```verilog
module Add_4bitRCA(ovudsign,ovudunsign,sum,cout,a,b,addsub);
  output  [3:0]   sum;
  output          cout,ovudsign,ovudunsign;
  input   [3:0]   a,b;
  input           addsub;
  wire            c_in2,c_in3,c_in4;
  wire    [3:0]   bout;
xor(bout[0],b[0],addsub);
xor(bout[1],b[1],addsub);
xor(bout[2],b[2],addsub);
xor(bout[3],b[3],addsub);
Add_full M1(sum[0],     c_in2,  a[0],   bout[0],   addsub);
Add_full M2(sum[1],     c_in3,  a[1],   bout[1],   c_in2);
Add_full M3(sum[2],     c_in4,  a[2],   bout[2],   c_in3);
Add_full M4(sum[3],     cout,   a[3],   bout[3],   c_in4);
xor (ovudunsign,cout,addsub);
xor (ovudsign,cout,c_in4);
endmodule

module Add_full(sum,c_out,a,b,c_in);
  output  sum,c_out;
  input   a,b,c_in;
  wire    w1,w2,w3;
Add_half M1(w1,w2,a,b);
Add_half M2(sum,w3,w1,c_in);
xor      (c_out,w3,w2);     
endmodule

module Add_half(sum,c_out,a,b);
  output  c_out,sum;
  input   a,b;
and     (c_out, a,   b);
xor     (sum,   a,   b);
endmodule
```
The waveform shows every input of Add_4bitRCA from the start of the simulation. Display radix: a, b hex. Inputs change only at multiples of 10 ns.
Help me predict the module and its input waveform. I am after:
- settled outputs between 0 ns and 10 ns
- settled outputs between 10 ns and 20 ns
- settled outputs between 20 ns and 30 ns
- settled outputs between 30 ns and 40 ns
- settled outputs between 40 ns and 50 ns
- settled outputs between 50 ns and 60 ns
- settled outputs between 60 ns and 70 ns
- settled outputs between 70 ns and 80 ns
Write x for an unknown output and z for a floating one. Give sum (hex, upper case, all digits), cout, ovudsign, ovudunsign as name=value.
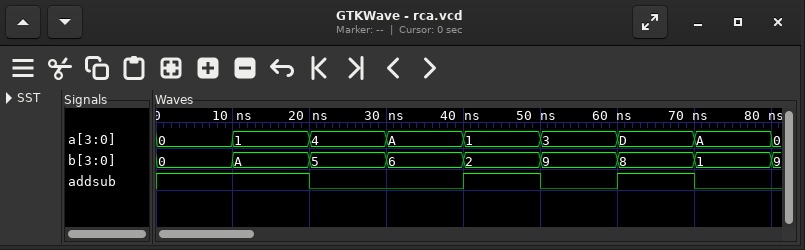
sum=0, cout=1, ovudsign=0, ovudunsign=0
sum=7, cout=0, ovudsign=0, ovudunsign=1
sum=9, cout=0, ovudsign=1, ovudunsign=0
sum=0, cout=1, ovudsign=0, ovudunsign=1
sum=F, cout=0, ovudsign=0, ovudunsign=1
sum=C, cout=0, ovudsign=0, ovudunsign=0
sum=5, cout=1, ovudsign=0, ovudunsign=0
sum=B, cout=0, ovudsign=0, ovudunsign=0
